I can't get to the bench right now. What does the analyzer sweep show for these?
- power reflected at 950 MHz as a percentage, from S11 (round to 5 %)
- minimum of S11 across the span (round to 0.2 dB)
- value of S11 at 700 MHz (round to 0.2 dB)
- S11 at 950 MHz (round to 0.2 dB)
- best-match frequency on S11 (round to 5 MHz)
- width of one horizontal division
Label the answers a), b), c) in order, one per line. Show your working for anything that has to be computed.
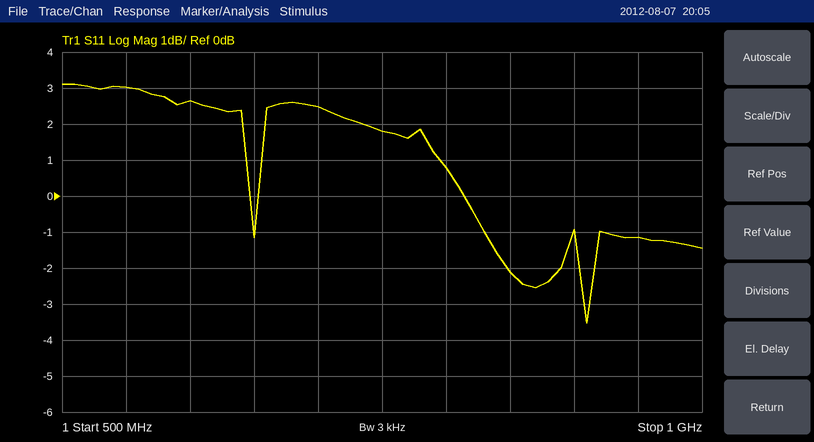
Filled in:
a) 10^(-1.2/10) ≈ 75.9 %, so 75 % to the nearest 5 %
b) -3.6 dB
c) 2.4 dB
d) -1.2 dB
e) 910 MHz
f) 50 MHz
